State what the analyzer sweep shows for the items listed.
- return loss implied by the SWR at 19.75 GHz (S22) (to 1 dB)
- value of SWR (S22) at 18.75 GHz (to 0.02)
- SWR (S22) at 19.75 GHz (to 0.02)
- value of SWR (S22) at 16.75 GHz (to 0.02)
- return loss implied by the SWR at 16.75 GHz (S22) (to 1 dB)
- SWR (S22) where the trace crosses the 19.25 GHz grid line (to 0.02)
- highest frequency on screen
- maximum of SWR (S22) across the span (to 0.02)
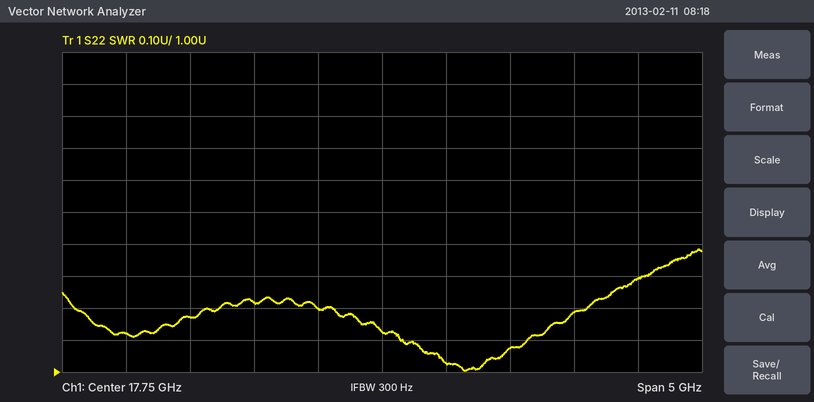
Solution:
18 dB
1.08
1.30
1.22
20 dB
1.18
20.25 GHz
1.38
